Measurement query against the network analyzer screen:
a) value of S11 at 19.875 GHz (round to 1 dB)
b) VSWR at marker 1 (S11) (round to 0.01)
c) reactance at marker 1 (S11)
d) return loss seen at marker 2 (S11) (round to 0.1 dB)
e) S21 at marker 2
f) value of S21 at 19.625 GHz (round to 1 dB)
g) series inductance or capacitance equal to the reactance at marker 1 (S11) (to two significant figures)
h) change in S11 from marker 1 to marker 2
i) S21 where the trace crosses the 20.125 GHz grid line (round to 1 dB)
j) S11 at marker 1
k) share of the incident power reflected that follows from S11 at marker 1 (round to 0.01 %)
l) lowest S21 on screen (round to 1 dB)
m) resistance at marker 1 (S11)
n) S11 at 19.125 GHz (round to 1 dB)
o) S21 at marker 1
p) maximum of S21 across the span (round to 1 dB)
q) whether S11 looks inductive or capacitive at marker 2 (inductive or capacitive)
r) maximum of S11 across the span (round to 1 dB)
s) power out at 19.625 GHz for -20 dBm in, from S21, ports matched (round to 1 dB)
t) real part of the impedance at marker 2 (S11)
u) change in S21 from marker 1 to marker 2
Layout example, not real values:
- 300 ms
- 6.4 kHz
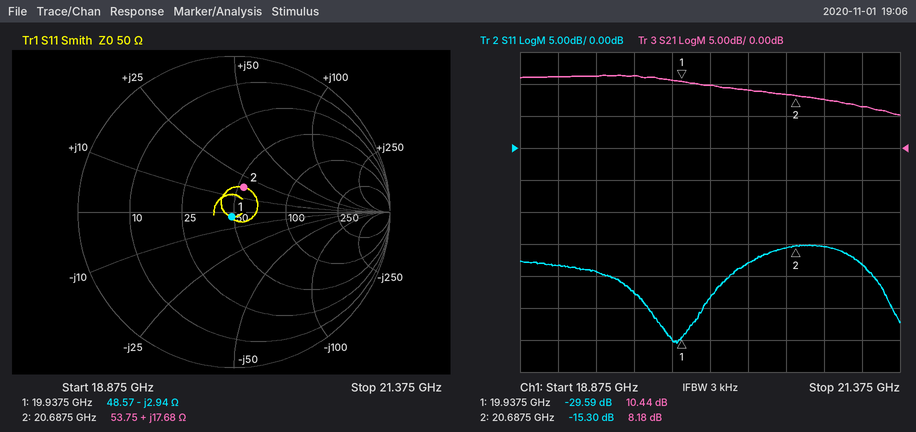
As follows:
- -30 dB
- 1.07
- -2.94 Ω
- 15.3 dB
- 8.18 dB
- 11 dB
- 2.7 pF
- 14.29 dB
- 10 dB
- -29.59 dB
- 0.11 %
- 5 dB
- 48.57 Ω
- -18 dB
- 10.44 dB
- 11 dB
- inductive
- -15 dB
- -9 dBm
- 53.75 Ω
- -2.26 dB
